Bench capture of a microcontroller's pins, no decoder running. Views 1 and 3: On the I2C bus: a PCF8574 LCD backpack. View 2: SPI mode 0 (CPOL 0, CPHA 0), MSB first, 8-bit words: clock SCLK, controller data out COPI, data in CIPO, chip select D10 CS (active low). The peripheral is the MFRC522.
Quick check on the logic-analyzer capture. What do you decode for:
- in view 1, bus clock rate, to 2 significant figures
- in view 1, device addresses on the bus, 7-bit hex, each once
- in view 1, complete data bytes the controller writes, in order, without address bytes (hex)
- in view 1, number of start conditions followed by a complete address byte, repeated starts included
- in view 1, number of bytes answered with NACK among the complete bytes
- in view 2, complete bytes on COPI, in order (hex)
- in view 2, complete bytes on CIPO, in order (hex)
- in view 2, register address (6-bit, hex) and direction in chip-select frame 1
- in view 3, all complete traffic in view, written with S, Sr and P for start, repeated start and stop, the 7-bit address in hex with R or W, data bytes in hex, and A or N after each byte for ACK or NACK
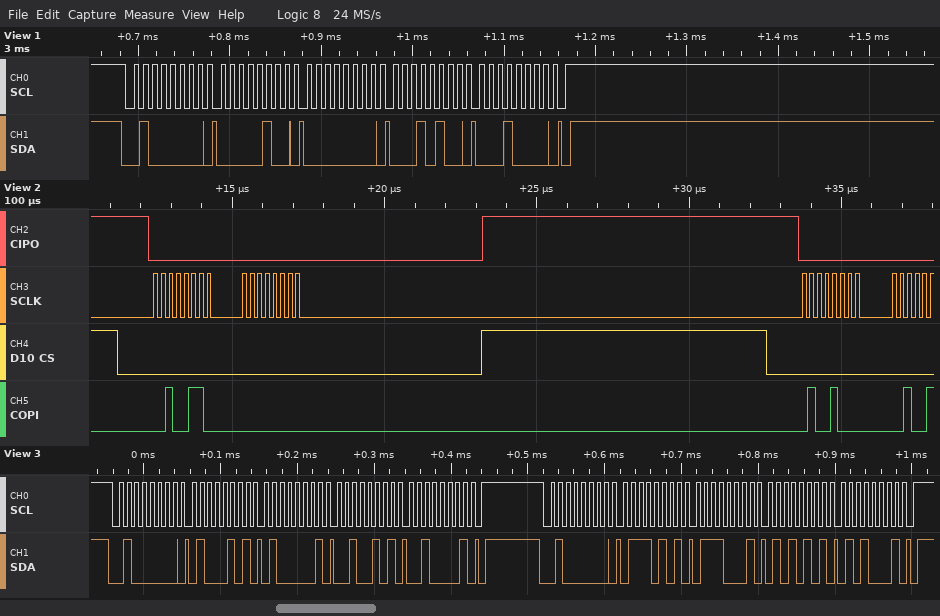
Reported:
100 kHz
0x20
04 00 14 10
1
0
0x26 0x00 0x48
0x00 0x00 0x00
0x13 write
S 20W A 45 A 41 A 25 A 21 A P S 20W A 75 A 71 A 55 A 51 A P
